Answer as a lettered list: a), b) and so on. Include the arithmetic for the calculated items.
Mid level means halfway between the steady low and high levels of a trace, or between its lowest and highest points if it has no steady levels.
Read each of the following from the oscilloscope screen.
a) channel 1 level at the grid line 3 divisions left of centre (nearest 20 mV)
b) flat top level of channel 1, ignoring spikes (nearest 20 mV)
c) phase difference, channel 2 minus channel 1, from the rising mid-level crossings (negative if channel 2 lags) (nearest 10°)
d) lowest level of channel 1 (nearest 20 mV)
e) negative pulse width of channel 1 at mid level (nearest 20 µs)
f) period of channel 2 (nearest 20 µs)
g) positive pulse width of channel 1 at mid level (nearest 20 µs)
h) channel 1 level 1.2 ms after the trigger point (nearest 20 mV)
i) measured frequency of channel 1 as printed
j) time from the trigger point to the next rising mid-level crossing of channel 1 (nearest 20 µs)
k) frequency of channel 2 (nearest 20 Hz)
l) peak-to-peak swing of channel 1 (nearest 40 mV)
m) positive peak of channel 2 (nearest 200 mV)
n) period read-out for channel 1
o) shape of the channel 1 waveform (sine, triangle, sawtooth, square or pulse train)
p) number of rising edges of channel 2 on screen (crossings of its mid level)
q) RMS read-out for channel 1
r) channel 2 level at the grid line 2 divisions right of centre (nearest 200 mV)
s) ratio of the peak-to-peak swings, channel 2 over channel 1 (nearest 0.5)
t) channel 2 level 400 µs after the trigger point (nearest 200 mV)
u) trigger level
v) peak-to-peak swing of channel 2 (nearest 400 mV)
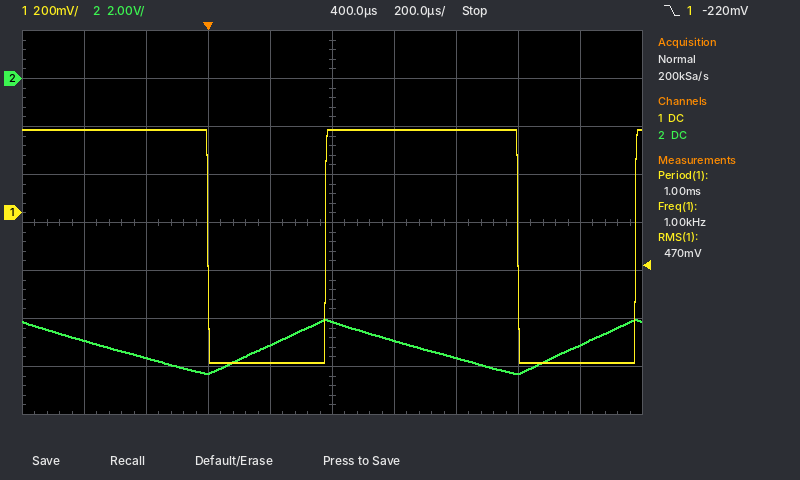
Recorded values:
a) 340 mV
b) 340 mV
c) +70°
d) -620 mV
e) 380 µs
f) 1.00 ms
g) 620 µs
h) -620 mV
i) 1.00 kHz
j) 380 µs
k) 1 / 1.00 ms ≈ 1.00 kHz
l) 960 mV
m) -10.0 V
n) 1.00 ms
o) pulse train
p) 2
q) 470 mV
r) -11.6 V
s) 2.4 V / 960 mV ≈ 2.5
t) -10.2 V
u) -220 mV
v) 2.4 V
